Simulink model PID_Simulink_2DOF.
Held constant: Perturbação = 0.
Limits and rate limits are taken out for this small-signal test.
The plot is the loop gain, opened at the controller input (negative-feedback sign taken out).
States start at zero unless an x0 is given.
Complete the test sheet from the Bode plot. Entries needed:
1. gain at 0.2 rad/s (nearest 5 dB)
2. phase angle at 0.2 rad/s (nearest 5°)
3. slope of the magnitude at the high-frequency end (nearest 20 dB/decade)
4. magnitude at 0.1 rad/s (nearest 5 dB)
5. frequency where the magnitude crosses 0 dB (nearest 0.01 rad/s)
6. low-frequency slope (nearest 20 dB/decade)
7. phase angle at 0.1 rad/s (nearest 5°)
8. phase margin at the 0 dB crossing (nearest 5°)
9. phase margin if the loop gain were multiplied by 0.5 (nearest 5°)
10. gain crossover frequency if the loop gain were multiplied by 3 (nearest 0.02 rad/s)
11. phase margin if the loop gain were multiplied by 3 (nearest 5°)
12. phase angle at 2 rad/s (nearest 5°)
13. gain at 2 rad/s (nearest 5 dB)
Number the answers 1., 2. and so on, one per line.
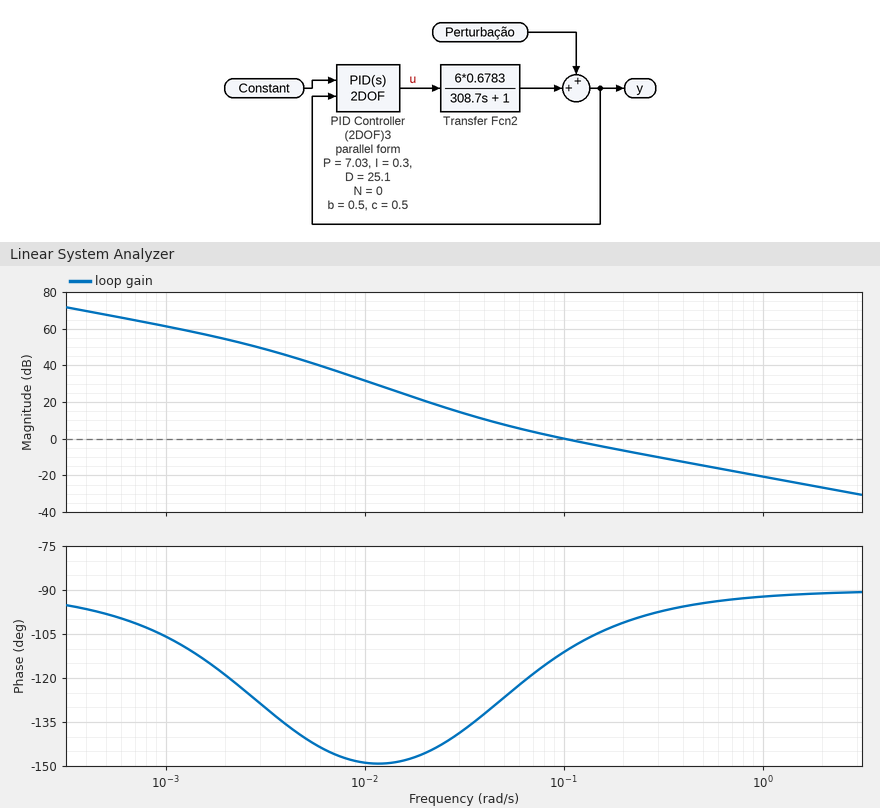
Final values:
1. -5 dB
2. -100°
3. -20 dB/decade
4. 0 dB
5. 0.10 rad/s
6. -20 dB/decade
7. -110°
8. 70°
9. 55°
10. 0.28 rad/s
11. 80°
12. -90°
13. -25 dB
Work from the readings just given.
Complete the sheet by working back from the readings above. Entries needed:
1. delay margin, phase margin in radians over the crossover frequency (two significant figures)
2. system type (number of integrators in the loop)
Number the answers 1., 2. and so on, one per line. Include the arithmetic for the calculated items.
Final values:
1. 70 × π / 180 / 0.1 = 12 s
2. 1
